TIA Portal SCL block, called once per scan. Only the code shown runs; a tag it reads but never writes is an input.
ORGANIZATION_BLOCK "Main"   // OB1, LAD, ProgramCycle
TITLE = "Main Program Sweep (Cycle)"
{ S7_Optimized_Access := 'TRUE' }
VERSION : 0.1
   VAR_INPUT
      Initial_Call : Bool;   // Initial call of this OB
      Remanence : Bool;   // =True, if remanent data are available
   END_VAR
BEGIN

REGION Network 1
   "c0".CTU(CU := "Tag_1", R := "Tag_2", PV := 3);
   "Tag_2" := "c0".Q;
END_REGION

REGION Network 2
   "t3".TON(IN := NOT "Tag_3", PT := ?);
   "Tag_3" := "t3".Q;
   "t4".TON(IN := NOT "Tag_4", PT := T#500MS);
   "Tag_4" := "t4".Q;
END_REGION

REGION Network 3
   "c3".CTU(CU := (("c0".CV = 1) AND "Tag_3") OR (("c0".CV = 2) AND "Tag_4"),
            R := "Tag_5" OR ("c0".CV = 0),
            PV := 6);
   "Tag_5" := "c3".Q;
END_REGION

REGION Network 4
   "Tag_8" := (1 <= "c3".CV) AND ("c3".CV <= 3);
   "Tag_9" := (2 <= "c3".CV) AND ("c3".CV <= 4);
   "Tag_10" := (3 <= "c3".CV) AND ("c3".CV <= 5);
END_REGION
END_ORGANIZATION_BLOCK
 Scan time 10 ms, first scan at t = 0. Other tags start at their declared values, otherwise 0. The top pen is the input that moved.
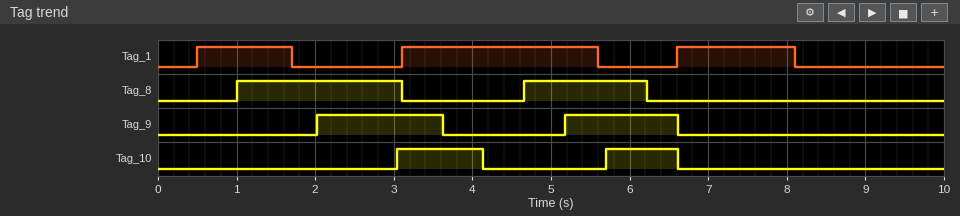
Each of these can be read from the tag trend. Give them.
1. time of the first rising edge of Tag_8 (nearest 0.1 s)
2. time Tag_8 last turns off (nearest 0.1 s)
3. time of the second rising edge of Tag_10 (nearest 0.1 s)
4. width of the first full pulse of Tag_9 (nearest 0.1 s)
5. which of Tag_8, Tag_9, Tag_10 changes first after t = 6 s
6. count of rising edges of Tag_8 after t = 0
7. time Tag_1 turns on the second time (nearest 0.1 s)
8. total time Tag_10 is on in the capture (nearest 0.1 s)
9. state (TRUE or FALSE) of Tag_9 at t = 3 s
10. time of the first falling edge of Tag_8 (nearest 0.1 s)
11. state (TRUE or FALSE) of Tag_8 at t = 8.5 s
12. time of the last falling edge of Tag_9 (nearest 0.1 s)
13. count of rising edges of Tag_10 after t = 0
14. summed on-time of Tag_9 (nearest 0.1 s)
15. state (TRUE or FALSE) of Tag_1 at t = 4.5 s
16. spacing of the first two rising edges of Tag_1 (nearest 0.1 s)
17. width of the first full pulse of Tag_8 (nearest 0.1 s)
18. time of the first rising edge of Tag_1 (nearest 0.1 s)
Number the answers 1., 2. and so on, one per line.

1. 1.0 s
2. 6.2 s
3. 5.7 s
4. 1.6 s
5. Tag_8
6. 2
7. 3.1 s
8. 2.0 s
9. TRUE
10. 3.1 s
11. FALSE
12. 6.6 s
13. 2
14. 3.0 s
15. TRUE
16. 2.6 s
17. 2.1 s
18. 0.5 s
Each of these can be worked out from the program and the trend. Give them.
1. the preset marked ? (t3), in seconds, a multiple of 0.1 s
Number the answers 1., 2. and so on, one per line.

1. 1.0 s
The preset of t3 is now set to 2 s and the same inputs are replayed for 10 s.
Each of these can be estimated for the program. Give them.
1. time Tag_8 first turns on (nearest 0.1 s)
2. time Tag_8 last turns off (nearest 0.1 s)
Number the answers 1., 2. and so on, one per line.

1. 2.0 s
2. 6.6 s
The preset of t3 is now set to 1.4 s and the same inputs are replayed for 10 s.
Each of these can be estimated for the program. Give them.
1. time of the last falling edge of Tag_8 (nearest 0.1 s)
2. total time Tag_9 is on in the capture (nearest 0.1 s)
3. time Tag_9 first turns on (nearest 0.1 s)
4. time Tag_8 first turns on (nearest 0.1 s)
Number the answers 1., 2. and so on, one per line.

1. 6.6 s
2. 2.2 s
3. 2.8 s
4. 1.4 s
